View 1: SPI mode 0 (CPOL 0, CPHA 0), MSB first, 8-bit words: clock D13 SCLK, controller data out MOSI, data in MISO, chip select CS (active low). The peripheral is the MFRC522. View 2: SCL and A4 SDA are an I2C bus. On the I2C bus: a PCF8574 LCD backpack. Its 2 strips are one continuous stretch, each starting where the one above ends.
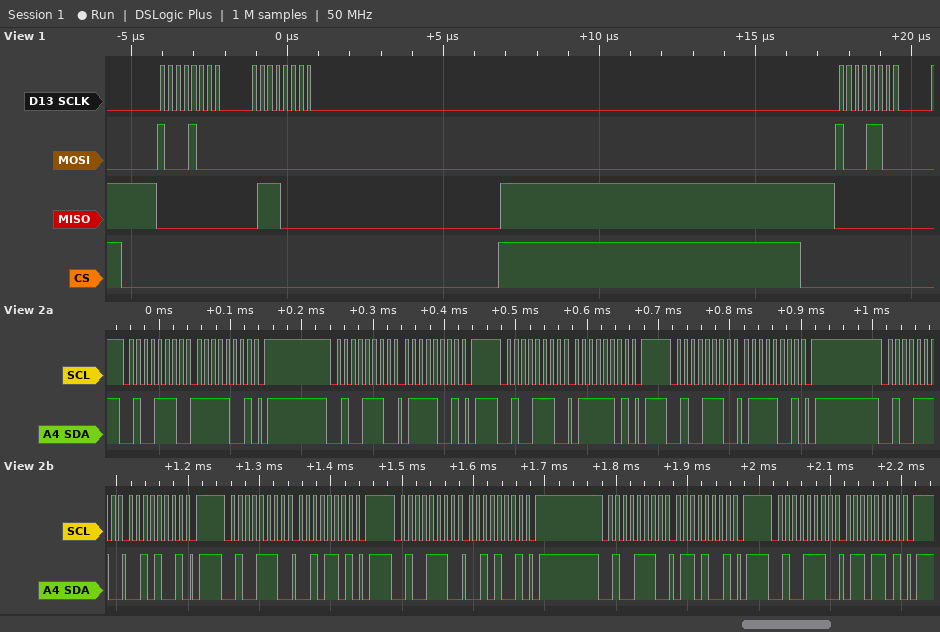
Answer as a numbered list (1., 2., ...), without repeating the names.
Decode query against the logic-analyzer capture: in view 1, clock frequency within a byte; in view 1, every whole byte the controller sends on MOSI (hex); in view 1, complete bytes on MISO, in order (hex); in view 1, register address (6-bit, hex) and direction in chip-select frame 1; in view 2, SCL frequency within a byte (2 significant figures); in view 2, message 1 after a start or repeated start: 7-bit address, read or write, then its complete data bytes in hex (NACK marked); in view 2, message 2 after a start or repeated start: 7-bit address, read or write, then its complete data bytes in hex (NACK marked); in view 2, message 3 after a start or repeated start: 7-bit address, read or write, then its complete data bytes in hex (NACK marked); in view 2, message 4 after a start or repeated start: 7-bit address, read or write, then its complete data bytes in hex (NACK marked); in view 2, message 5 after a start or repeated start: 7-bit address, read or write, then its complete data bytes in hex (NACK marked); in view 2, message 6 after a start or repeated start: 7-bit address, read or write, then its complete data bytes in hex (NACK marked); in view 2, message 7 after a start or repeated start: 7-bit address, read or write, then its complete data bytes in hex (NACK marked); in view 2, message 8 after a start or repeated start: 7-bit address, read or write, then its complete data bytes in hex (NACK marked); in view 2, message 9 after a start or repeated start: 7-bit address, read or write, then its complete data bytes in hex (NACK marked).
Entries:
1. 4 MHz
2. 88 00 8C
3. 00 70 00
4. 0x04 read
5. 100 kHz
6. 0x27 write: F9
7. 0x27 write: 79
8. 0x27 write: 7D
9. 0x27 write: 79
10. 0x27 write: 29
11. 0x27 write: 2D
12. 0x27 write: 29
13. 0x27 write: 69
14. 0x27 write: 6D
